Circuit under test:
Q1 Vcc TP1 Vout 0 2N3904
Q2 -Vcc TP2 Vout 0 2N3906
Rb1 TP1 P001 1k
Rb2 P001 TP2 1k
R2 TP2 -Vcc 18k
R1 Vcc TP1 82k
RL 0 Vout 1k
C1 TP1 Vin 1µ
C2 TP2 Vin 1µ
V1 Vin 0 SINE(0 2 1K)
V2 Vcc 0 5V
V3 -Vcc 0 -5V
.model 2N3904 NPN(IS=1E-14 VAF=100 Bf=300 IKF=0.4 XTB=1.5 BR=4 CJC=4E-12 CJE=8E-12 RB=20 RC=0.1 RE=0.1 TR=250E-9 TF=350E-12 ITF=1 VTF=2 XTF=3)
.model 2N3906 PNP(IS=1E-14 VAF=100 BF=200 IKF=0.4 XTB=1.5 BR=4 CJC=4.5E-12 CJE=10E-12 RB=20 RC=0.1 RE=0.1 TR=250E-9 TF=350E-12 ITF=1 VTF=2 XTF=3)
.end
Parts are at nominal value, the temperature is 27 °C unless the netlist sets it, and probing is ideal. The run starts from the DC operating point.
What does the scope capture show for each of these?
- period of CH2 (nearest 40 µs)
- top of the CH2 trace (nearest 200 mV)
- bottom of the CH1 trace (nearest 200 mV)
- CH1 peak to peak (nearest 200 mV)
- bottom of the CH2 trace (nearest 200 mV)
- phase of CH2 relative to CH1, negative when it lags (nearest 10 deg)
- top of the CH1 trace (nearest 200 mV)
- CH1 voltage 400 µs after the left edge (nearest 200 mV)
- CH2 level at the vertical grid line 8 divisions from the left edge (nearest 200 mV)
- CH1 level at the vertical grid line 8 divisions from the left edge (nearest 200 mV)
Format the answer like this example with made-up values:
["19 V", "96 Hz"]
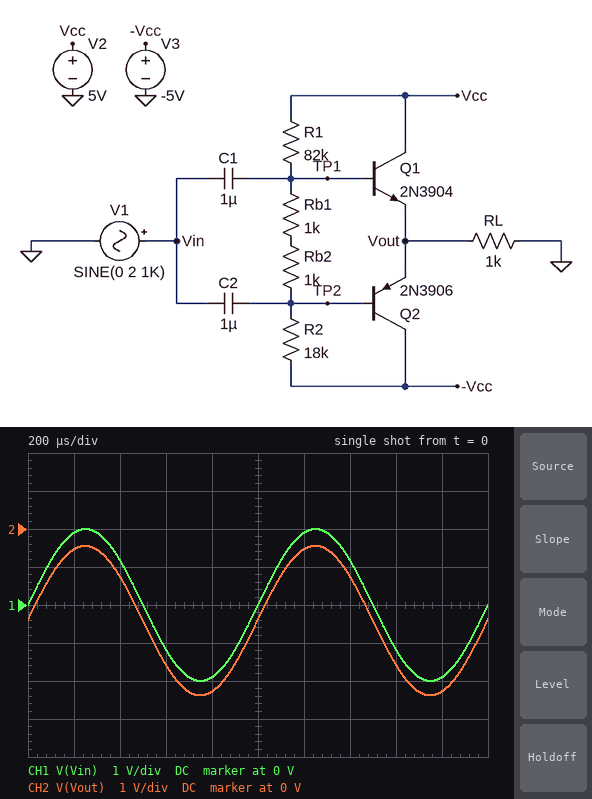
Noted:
["1.00 ms", "-400 mV", "-2.0 V", "4.0 V", "-4.4 V", "0 deg", "2.0 V", "1.2 V", "-3.6 V", "-1.2 V"]
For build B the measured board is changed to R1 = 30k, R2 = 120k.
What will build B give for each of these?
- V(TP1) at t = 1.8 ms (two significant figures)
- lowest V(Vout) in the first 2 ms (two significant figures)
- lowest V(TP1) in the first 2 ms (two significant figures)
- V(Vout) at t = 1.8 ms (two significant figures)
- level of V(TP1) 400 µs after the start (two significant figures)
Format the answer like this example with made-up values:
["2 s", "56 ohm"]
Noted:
["950 mV", "230 mV", "850 mV", "320 mV", "4.0 V"]
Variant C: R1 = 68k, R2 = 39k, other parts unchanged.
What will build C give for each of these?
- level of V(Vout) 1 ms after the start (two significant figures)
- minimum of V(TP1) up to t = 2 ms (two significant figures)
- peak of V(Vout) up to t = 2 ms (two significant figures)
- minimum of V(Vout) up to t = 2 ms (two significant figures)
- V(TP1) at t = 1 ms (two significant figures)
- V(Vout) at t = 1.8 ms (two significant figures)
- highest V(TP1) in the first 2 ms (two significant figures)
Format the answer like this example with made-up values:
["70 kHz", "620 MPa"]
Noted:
["-690 mV", "-3.2 V", "220 mV", "-2.7 V", "-1.2 V", "-2.6 V", "840 mV"]
